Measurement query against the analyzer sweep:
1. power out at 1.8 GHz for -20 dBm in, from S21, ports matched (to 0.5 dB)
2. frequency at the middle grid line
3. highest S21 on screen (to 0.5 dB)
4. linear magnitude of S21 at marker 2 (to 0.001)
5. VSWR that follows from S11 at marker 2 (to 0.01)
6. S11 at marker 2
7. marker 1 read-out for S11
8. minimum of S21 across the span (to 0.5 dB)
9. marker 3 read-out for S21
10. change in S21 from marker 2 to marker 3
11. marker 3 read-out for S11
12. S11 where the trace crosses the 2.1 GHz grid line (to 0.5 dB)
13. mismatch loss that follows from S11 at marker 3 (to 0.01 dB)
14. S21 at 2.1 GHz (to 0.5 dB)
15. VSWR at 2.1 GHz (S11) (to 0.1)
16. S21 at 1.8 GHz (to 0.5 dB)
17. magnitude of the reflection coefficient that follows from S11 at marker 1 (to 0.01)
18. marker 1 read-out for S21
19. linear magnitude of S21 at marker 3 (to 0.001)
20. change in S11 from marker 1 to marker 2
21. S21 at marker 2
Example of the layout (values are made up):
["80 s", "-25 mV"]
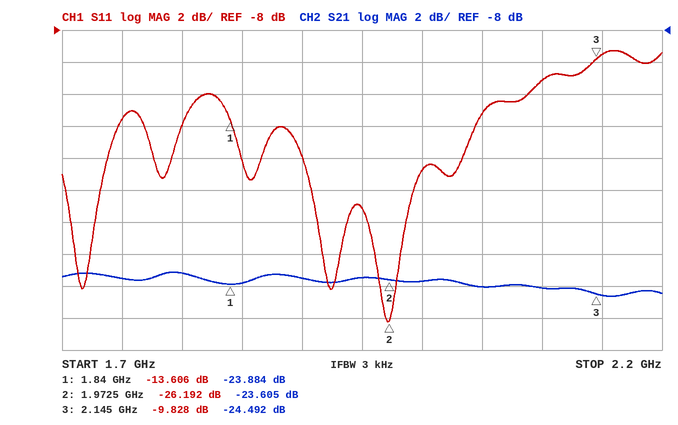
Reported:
["-43.0 dBm", "1.95 GHz", "-23.0 dB", "0.066", "1.10", "-26.192 dB", "-13.606 dB", "-24.5 dB", "-24.492 dB", "-0.887 dB", "-9.828 dB", "-11.0 dB", "0.48 dB", "-24.0 dB", "1.8", "-23.0 dB", "0.21", "-23.884 dB", "0.060", "-12.586 dB", "-23.605 dB"]
